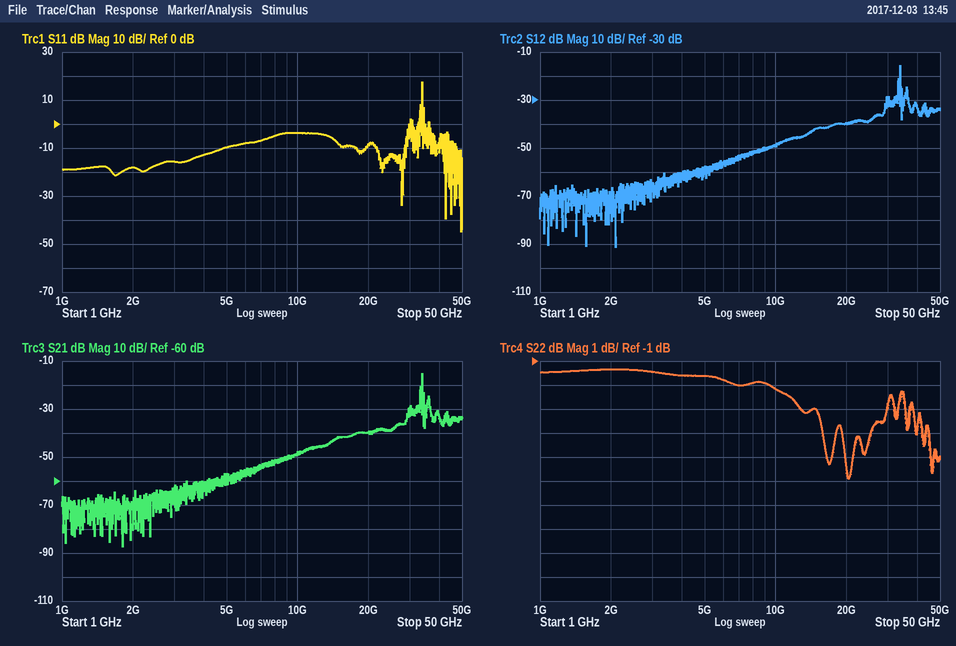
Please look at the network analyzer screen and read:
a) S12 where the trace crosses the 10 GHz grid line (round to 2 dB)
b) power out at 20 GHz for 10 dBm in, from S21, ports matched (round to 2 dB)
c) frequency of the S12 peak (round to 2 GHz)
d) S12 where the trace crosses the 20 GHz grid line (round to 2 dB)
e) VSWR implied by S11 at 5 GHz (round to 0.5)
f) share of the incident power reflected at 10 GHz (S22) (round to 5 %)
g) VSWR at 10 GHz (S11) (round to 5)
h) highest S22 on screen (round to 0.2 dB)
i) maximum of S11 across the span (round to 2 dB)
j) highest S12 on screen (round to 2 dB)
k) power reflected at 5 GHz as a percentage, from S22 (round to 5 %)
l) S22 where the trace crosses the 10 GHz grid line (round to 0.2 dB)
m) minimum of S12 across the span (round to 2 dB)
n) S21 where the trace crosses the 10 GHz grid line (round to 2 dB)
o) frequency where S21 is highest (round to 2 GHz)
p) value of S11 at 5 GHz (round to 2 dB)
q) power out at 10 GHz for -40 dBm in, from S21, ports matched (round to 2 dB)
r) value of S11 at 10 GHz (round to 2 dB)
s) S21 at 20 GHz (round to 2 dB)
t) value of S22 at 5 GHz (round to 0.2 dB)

-48 dB
-30 dBm
34 GHz
-40 dB
2.0
60 %
5
-1.4 dB
18 dB
-16 dB
70 %
-2.2 dB
-92 dB
-48 dB
34 GHz
-10 dB
-88 dBm
-4 dB
-40 dB
-1.6 dB
